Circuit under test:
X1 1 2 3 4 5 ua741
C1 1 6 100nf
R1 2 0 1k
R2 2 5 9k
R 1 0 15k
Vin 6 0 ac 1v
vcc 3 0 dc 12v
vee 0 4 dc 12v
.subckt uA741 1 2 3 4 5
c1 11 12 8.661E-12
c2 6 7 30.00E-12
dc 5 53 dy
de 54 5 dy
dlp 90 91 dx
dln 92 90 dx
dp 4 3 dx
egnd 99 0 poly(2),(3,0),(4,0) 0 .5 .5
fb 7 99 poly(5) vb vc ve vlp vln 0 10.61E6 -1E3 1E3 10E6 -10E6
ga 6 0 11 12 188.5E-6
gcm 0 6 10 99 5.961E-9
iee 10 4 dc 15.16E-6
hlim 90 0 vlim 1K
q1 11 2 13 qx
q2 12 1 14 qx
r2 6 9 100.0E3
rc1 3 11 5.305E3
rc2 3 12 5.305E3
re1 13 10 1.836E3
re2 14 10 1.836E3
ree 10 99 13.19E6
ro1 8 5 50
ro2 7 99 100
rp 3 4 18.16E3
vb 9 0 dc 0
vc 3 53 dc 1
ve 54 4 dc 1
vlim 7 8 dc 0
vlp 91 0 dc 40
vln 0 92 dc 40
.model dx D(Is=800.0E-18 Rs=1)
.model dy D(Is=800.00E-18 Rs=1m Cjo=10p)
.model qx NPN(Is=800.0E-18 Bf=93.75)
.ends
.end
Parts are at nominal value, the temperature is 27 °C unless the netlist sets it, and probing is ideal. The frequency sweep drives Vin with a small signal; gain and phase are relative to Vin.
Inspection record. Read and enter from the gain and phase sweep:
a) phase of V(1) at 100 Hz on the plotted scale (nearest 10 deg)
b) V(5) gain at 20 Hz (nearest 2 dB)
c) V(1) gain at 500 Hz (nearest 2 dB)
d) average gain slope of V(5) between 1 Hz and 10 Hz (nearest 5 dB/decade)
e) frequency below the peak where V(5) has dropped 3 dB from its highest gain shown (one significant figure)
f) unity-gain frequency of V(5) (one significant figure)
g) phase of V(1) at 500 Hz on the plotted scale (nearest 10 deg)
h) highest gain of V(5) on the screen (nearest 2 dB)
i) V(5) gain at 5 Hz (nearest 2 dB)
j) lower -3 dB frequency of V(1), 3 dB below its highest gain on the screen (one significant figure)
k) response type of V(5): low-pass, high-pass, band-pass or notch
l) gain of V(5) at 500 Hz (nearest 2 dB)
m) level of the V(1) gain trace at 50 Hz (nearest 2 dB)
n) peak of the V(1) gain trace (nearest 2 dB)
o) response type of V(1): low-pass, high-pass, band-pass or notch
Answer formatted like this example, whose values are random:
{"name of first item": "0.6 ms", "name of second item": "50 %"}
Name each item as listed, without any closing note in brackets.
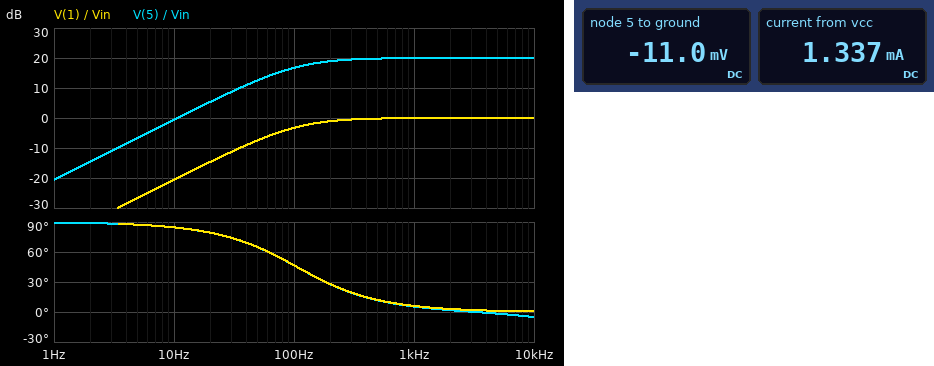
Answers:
{"phase of V(1) at 100 Hz on the plotted scale": "50 deg", "V(5) gain at 20 Hz": "6 dB", "V(1) gain at 500 Hz": "0 dB", "average gain slope of V(5) between 1 Hz and 10 Hz": "20 dB/decade", "frequency below the peak where V(5) has dropped 3 dB from its highest gain shown": "100 Hz", "unity-gain frequency of V(5)": "10 Hz", "phase of V(1) at 500 Hz on the plotted scale": "10 deg", "highest gain of V(5) on the screen": "20 dB", "V(5) gain at 5 Hz": "-6 dB", "lower -3 dB frequency of V(1), 3 dB below its highest gain on the screen": "100 Hz", "response type of V(5): low-pass, high-pass, band-pass or notch": "high-pass", "gain of V(5) at 500 Hz": "20 dB", "level of the V(1) gain trace at 50 Hz": "-8 dB", "peak of the V(1) gain trace": "0 dB", "response type of V(1): low-pass, high-pass, band-pass or notch": "high-pass"}
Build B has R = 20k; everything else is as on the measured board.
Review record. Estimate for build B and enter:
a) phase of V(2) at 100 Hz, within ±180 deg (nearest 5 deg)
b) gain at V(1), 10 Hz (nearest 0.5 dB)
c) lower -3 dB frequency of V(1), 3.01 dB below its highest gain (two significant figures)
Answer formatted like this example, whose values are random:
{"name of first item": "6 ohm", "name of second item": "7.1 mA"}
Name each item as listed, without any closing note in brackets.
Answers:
{"phase of V(2) at 100 Hz, within ±180 deg": "40 deg", "gain at V(1), 10 Hz": "-18.0 dB", "lower -3 dB frequency of V(1), 3.01 dB below its highest gain": "80 Hz"}
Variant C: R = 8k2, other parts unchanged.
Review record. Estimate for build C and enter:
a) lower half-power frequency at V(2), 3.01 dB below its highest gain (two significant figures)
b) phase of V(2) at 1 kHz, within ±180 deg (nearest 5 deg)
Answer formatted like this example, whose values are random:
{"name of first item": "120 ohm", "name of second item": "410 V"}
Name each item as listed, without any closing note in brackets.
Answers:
{"lower half-power frequency at V(2), 3.01 dB below its highest gain": "190 Hz", "phase of V(2) at 1 kHz, within ±180 deg": "10 deg"}
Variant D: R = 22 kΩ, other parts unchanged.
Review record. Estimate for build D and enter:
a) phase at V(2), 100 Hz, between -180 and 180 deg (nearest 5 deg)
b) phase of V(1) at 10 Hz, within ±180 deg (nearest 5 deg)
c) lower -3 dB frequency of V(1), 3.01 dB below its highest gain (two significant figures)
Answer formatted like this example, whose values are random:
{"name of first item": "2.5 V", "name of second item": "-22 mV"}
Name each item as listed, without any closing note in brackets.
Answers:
{"phase at V(2), 100 Hz, between -180 and 180 deg": "35 deg", "phase of V(1) at 10 Hz, within ±180 deg": "80 deg", "lower -3 dB frequency of V(1), 3.01 dB below its highest gain": "72 Hz"}
